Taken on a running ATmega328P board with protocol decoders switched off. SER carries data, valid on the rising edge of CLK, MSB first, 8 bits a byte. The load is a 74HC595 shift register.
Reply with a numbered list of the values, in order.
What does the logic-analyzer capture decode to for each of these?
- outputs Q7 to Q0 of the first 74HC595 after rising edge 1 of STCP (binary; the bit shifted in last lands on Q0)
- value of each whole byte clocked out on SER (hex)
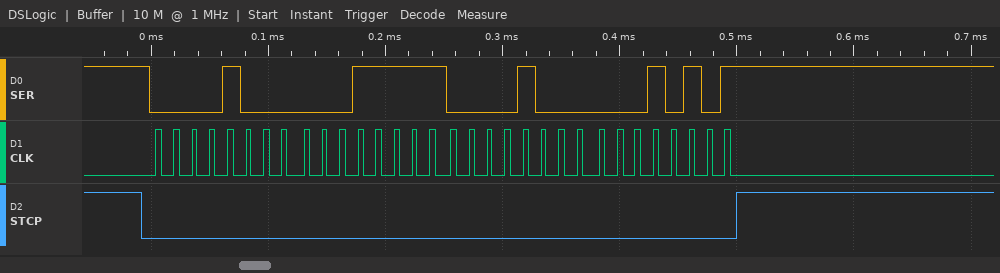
1. 00010101
2. 08 1F 08 15
